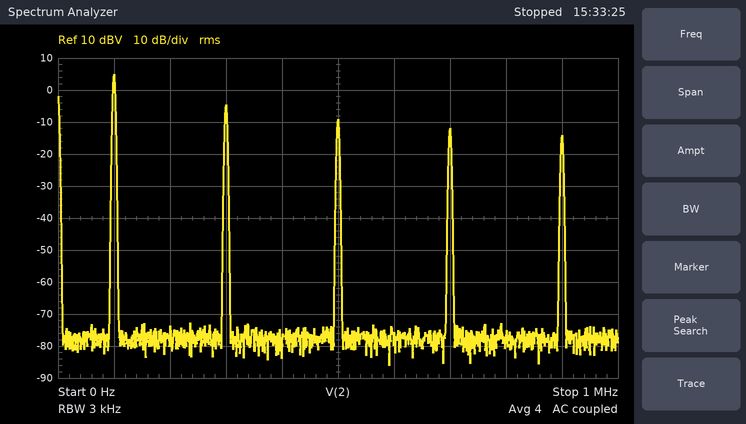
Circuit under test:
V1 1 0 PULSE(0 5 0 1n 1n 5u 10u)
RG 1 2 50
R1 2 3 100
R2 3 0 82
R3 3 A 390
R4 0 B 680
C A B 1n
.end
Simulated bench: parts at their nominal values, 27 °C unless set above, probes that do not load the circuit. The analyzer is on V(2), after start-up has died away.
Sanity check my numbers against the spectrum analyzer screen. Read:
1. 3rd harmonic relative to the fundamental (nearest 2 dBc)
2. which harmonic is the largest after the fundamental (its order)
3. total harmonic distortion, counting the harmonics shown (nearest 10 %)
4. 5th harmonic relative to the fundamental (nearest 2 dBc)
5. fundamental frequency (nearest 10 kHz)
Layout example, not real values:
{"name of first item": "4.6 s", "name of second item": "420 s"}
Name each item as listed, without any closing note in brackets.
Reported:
{"3rd harmonic relative to the fundamental": "-10 dBc", "which harmonic is the largest after the fundamental": "3", "total harmonic distortion, counting the harmonics shown": "40 %", "5th harmonic relative to the fundamental": "-14 dBc", "fundamental frequency": "100 kHz"}
